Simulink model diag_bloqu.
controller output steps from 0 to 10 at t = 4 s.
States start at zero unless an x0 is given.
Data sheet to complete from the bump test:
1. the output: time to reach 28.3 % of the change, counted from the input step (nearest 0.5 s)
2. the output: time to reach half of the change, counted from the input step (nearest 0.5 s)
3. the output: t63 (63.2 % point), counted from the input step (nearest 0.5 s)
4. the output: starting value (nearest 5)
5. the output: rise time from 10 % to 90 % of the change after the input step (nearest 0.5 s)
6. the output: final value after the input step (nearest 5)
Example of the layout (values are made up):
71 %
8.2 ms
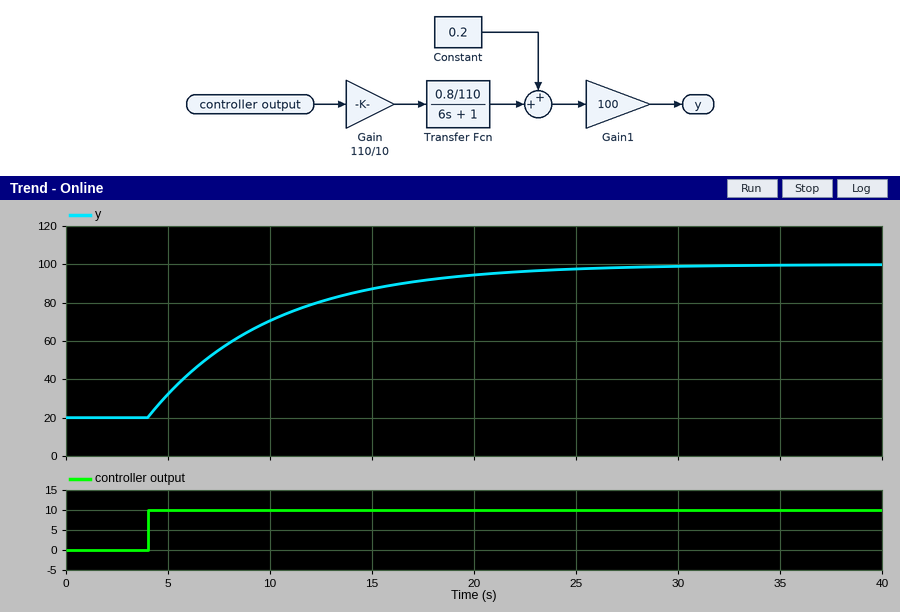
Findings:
2.0 s
4.0 s
6.0 s
20
13.0 s
100
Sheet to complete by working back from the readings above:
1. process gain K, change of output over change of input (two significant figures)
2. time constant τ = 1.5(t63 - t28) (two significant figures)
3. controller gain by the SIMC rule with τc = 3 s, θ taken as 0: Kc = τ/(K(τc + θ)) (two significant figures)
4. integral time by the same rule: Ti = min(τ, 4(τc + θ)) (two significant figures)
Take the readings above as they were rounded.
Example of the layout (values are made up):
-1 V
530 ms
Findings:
8.0
6.0 s
0.25
6.0 s
